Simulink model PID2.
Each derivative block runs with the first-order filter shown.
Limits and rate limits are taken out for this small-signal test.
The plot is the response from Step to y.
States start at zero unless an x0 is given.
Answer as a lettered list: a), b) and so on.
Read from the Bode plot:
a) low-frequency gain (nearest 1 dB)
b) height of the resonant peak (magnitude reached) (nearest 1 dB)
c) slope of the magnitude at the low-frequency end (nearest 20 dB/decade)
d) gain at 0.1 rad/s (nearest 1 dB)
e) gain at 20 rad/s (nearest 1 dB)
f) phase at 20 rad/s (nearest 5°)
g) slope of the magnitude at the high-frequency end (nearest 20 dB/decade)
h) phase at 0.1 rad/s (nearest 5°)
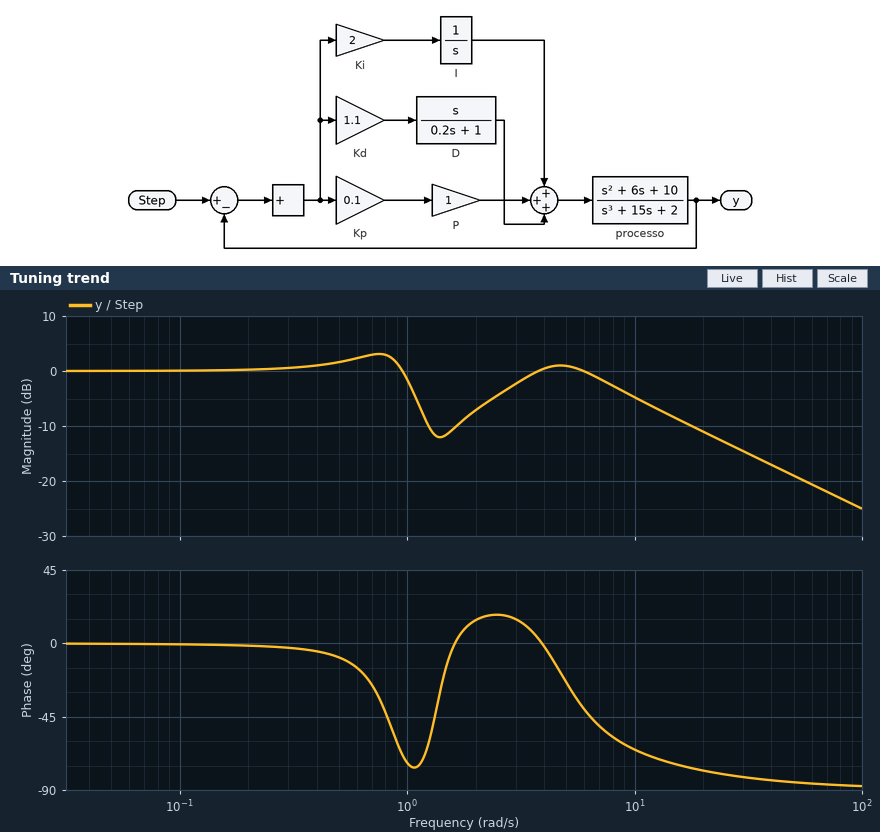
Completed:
a) 0 dB
b) 3 dB
c) 0 dB/decade
d) 0 dB
e) -11 dB
f) -80°
g) -20 dB/decade
h) 0°
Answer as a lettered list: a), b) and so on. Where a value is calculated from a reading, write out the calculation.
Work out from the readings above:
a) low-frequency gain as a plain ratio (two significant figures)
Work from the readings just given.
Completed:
a) 10^(0 / 20) = 1.0
